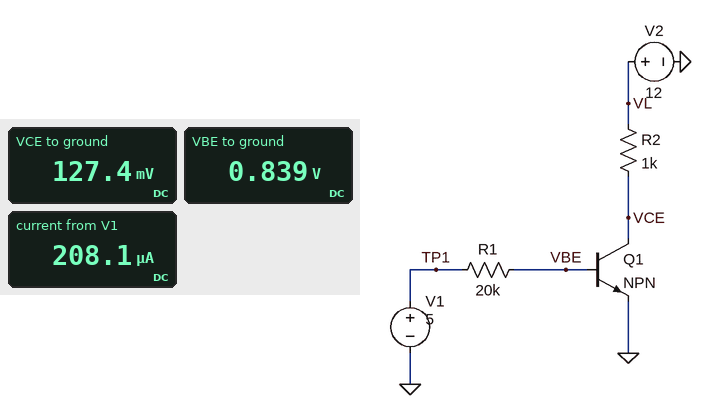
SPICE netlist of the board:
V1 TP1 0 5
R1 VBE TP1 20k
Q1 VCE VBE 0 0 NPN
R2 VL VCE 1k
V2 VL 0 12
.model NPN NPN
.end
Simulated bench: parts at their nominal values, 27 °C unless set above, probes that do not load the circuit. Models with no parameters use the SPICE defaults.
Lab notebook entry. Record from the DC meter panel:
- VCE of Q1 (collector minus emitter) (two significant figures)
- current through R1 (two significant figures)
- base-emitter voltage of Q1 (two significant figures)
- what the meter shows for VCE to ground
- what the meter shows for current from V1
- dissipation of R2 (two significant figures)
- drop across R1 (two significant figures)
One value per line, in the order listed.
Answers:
130 mV
210 µA
840 mV
127.4 mV
208.1 µA
140 mW
4.2 V
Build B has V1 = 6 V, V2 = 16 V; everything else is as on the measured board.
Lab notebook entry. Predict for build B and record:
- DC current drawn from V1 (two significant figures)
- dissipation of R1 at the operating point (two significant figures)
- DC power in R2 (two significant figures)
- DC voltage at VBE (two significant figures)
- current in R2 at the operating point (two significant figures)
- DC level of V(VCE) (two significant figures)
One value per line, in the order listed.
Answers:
260 µA
1.3 mW
250 mW
850 mV
16 mA
130 mV
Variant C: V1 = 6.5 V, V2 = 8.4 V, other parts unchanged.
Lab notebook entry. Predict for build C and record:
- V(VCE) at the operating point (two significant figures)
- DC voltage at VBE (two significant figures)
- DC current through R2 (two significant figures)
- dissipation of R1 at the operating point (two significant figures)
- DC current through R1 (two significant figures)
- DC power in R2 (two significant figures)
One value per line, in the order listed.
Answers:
98 mV
830 mV
8.3 mA
1.6 mW
280 µA
69 mW
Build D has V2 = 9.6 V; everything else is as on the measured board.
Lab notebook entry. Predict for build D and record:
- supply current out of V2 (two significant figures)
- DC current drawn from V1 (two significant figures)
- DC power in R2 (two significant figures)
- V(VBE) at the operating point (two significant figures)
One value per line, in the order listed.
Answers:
9.5 mA
210 µA
90 mW
830 mV
